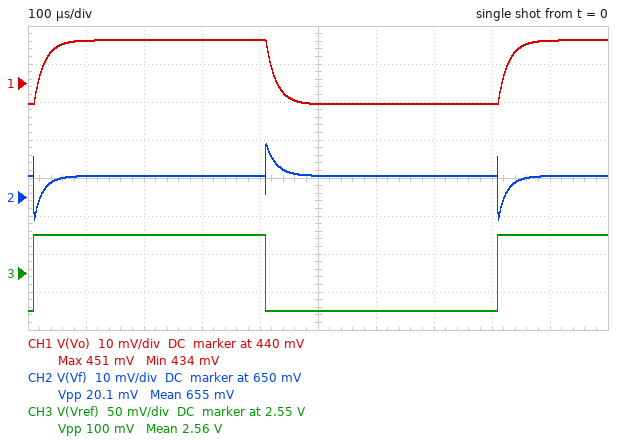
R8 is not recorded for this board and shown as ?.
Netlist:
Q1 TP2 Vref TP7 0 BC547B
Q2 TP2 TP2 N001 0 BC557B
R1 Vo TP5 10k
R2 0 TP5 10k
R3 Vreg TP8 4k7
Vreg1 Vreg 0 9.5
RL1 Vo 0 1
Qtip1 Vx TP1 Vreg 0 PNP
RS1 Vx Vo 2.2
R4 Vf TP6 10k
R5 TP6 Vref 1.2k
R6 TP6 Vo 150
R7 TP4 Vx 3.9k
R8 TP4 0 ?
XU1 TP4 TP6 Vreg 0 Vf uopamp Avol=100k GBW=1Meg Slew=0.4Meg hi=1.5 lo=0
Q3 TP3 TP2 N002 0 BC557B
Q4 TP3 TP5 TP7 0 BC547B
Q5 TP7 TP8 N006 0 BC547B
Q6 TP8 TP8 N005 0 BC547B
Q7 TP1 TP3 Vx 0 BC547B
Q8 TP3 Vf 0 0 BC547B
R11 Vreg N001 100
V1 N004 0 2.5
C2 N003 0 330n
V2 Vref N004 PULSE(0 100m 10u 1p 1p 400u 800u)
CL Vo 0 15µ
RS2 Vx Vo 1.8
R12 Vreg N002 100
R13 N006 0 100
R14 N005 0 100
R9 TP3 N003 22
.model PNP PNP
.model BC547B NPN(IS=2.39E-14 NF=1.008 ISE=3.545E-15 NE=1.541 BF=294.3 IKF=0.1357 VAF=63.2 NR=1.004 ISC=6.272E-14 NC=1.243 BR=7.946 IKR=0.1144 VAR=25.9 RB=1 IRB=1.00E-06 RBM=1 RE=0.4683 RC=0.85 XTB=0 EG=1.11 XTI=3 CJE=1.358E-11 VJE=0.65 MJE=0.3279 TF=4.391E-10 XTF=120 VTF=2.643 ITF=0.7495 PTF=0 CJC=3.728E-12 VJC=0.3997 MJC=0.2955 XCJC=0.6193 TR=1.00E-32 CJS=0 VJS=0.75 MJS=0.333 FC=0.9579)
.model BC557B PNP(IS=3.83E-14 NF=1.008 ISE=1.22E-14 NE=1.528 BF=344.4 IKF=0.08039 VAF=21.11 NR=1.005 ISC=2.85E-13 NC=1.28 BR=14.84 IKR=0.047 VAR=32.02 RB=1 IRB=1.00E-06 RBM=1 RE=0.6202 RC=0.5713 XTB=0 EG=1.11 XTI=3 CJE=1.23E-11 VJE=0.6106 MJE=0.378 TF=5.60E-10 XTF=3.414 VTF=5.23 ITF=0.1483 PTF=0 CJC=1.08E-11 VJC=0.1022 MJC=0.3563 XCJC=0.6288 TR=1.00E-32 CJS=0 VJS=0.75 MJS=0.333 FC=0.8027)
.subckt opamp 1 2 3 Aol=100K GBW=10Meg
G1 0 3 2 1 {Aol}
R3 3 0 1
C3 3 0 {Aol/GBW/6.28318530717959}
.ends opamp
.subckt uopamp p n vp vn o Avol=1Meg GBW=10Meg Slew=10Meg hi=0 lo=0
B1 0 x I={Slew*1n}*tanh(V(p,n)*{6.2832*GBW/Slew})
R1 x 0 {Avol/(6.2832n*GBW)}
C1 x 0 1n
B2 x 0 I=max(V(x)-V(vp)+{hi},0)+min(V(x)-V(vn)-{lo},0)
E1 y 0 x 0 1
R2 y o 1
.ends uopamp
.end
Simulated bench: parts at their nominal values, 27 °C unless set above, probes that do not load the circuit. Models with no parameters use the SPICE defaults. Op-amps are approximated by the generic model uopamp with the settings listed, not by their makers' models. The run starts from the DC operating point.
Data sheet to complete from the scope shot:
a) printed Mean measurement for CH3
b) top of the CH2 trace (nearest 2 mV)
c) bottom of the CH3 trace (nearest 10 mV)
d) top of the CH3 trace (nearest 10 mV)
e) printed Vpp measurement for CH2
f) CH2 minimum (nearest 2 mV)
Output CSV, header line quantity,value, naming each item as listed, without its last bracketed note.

quantity,value
printed Mean measurement for CH3,2.56 V
top of the CH2 trace,664 mV
bottom of the CH3 trace,2.50 V
top of the CH3 trace,2.60 V
printed Vpp measurement for CH2,20.1 mV
CH2 minimum,644 mV
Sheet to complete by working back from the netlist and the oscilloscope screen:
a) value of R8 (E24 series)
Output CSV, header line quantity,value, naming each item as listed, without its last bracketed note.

quantity,value
value of R8,13 kΩ
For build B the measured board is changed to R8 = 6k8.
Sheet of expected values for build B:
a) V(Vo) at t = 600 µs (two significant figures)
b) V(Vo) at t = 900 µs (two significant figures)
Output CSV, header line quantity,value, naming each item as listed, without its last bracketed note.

quantity,value
V(Vo) at t = 600 µs,730 mV
V(Vo) at t = 900 µs,760 mV
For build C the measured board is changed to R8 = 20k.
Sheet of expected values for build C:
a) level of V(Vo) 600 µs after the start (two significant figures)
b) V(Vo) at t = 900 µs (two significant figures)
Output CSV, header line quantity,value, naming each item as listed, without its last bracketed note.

quantity,value
level of V(Vo) 600 µs after the start,360 mV
V(Vo) at t = 900 µs,370 mV
